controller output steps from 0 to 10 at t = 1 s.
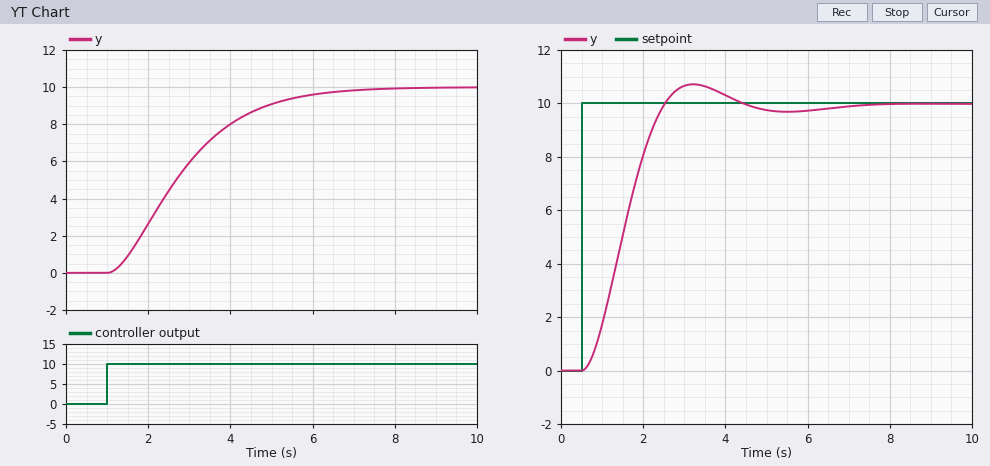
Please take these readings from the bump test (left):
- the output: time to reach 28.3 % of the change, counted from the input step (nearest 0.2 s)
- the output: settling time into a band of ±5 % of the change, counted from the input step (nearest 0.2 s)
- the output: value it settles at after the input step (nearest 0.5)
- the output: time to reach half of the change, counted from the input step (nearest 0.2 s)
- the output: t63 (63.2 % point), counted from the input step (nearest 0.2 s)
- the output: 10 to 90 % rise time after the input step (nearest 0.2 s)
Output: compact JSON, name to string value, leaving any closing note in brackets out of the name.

{"the output: time to reach 28.3 % of the change, counted from the input step": "1.0 s", "the output: settling time into a band of ±5 % of the change, counted from the input step": "4.8 s", "the output: value it settles at after the input step": "10.0", "the output: time to reach half of the change, counted from the input step": "1.6 s", "the output: t63 (63.2 % point), counted from the input step": "2.2 s", "the output: 10 to 90 % rise time after the input step": "3.4 s"}
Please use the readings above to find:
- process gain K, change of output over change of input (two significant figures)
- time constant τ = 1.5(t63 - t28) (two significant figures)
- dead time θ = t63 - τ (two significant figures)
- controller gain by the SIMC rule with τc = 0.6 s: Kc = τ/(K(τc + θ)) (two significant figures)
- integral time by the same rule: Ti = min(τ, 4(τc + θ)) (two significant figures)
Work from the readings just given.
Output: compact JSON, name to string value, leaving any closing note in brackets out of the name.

{"process gain K, change of output over change of input": "1.0", "time constant τ = 1.5(t63 - t28)": "1.8 s", "dead time θ = t63 - τ": "0.40 s", "controller gain by the SIMC rule with τc = 0.6 s: Kc = τ/(K(τc + θ))": "1.8", "integral time by the same rule: Ti = min(τ, 4(τc + θ))": "1.8 s"}
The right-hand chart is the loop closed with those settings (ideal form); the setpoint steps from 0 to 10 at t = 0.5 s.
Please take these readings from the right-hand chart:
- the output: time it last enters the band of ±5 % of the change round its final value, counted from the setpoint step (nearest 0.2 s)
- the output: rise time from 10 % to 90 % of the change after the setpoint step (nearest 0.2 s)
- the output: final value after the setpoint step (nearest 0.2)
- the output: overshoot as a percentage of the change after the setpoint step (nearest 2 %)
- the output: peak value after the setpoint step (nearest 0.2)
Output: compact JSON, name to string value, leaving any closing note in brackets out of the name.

{"the output: time it last enters the band of ±5 % of the change round its final value, counted from the setpoint step": "3.2 s", "the output: rise time from 10 % to 90 % of the change after the setpoint step": "1.4 s", "the output: final value after the setpoint step": "10.0", "the output: overshoot as a percentage of the change after the setpoint step": "8 %", "the output: peak value after the setpoint step": "10.8"}
